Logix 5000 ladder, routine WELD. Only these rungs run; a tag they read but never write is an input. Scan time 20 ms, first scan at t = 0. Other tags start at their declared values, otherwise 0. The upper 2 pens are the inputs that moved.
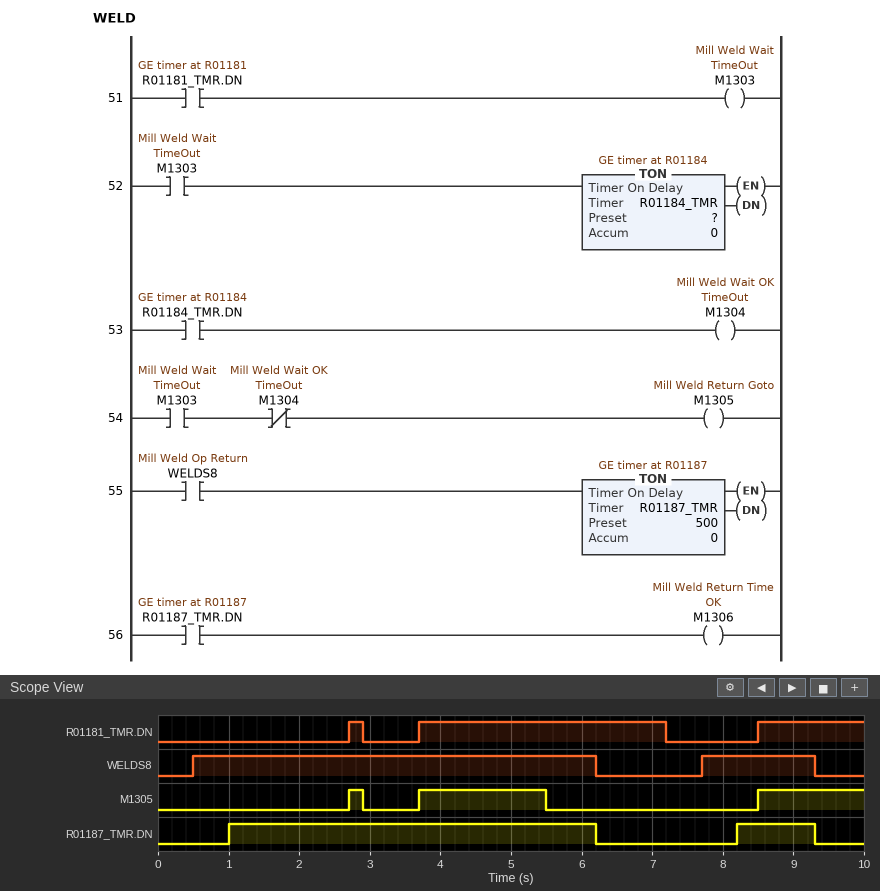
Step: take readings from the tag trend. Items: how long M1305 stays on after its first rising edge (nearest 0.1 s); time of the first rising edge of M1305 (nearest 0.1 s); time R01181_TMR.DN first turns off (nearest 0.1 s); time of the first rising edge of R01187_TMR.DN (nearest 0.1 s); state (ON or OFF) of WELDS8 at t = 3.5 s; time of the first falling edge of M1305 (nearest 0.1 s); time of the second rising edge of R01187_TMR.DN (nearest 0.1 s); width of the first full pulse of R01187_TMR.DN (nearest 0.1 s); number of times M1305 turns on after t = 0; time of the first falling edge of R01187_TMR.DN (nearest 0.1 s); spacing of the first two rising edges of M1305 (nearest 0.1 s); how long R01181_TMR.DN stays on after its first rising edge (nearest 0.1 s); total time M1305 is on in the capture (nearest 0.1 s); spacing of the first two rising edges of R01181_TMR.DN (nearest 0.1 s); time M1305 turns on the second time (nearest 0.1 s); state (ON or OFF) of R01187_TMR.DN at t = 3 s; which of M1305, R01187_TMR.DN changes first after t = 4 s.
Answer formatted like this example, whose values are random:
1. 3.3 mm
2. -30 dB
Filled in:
1. 0.2 s
2. 2.7 s
3. 2.9 s
4. 1.0 s
5. ON
6. 2.9 s
7. 8.2 s
8. 5.2 s
9. 3
10. 6.2 s
11. 1.0 s
12. 0.2 s
13. 3.5 s
14. 1.0 s
15. 3.7 s
16. ON
17. M1305
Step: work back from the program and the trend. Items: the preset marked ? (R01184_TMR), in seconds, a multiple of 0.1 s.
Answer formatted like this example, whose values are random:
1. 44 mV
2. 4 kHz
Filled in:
1. 1.8 s
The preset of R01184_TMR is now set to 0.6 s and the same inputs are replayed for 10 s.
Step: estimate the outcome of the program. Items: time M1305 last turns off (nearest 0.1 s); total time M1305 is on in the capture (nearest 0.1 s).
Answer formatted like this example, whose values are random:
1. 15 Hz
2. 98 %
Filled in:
1. 9.1 s
2. 1.4 s
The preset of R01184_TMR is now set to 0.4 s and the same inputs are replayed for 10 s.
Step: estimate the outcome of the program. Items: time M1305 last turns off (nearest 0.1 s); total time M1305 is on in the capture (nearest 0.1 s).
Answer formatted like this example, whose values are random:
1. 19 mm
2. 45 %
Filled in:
1. 8.9 s
2. 1.0 s
